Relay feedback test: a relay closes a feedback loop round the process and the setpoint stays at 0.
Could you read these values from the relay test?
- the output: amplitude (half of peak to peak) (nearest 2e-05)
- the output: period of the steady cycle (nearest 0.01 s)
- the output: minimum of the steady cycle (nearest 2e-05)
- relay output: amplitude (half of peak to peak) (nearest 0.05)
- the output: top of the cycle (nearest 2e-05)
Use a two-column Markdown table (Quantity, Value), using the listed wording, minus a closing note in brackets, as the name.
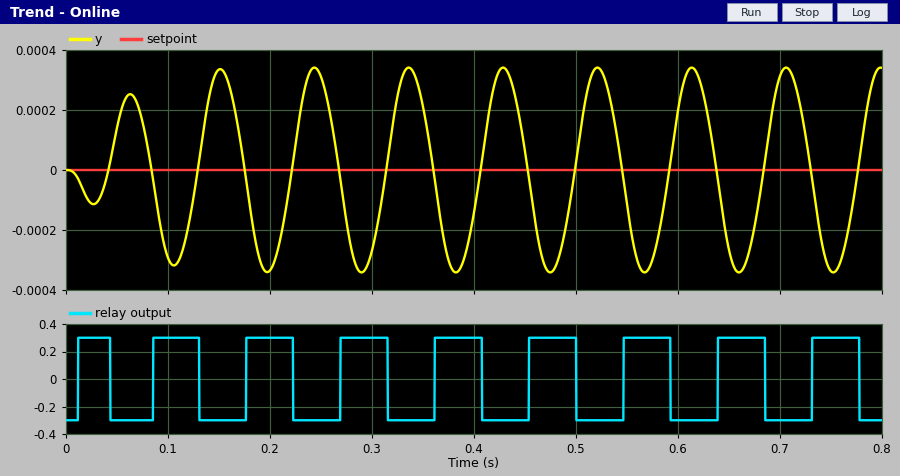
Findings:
| Quantity | Value |
|---|---|
| the output: amplitude (half of peak to peak) | 0.00034 |
| the output: period of the steady cycle | 0.09 s |
| the output: minimum of the steady cycle | -0.00034 |
| relay output: amplitude (half of peak to peak) | 0.30 |
| the output: top of the cycle | 0.00034 |
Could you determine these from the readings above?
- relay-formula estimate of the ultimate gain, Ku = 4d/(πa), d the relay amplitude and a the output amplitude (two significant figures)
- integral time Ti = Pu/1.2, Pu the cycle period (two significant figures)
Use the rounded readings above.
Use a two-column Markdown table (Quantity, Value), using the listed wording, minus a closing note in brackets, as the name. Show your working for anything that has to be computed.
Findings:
| Quantity | Value |
|---|---|
| relay-formula estimate of the ultimate gain, Ku = 4d/(πa), d the relay amplitude and a the output amplitude | 4 × 0.3 / (π × 0.00034) = 1100 |
| integral time Ti = Pu/1.2, Pu the cycle period | 0.09 / 1.2 = 0.075 s |
